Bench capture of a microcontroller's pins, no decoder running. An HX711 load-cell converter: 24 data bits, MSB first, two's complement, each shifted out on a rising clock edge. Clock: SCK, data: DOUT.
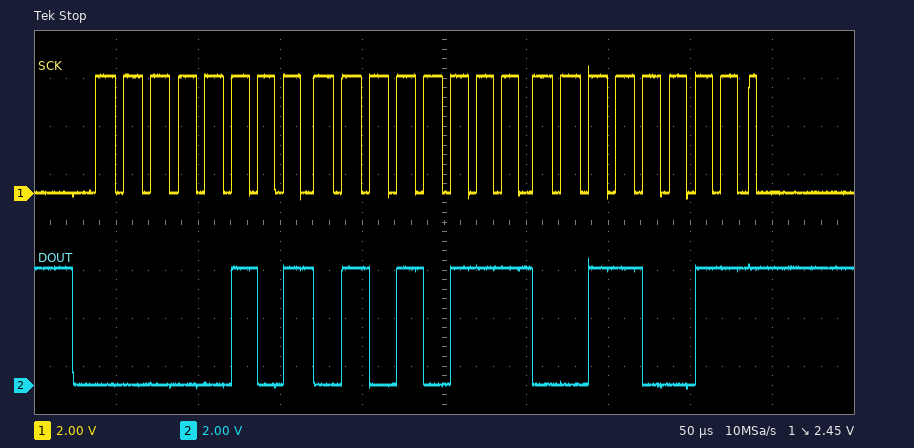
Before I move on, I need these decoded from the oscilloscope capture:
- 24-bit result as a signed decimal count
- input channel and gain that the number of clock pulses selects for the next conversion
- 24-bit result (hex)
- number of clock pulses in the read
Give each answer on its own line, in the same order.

350003
channel A, gain 128
0x055733
25
